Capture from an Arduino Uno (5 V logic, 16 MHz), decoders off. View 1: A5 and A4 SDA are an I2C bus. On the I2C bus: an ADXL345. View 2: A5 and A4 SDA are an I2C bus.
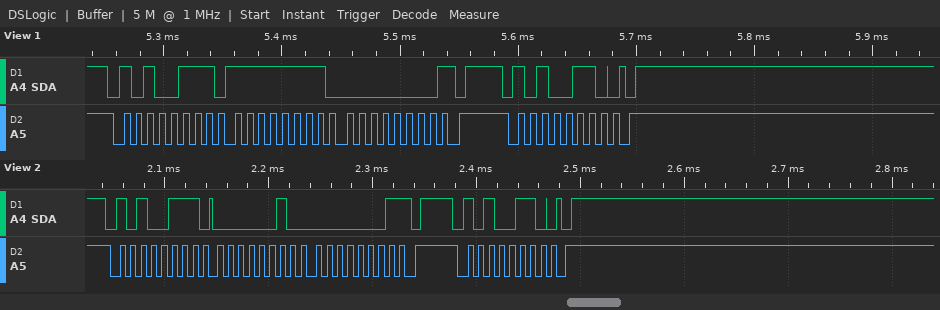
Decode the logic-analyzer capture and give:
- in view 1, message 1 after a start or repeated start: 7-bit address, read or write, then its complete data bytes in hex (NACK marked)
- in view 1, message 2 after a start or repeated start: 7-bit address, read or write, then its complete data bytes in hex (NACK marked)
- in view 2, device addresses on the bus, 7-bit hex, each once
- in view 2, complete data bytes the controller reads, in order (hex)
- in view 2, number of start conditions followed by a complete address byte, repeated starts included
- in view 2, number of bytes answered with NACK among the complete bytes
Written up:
0x53 read: FF 00 NACK
0x53 write
0x53
02 01
2
1
